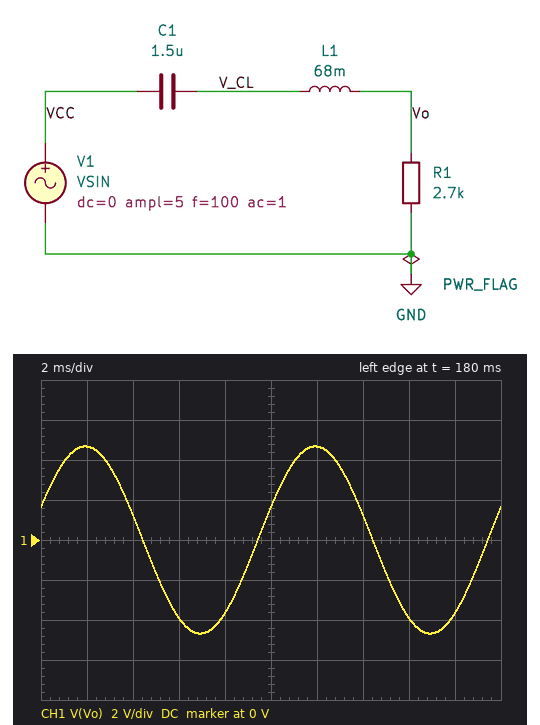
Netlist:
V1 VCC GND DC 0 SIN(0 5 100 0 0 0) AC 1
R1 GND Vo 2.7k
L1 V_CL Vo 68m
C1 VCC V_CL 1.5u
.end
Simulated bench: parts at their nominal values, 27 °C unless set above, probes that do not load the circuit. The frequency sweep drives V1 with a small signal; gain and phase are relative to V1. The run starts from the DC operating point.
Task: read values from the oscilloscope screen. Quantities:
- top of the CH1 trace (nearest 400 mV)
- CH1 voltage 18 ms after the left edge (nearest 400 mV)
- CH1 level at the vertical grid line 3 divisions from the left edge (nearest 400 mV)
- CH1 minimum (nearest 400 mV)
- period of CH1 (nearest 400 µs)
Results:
4.8 V
-3.6 V
-4.0 V
-4.8 V
10.0 ms
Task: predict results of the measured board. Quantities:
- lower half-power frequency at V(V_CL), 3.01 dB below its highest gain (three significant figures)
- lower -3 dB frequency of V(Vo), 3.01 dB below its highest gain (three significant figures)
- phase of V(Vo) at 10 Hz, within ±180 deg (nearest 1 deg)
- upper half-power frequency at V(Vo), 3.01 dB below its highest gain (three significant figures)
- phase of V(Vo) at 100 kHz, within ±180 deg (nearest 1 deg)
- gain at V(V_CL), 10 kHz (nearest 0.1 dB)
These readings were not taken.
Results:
39.5 Hz
39.1 Hz
76 deg
6.36 kHz
-86 deg
0 dB
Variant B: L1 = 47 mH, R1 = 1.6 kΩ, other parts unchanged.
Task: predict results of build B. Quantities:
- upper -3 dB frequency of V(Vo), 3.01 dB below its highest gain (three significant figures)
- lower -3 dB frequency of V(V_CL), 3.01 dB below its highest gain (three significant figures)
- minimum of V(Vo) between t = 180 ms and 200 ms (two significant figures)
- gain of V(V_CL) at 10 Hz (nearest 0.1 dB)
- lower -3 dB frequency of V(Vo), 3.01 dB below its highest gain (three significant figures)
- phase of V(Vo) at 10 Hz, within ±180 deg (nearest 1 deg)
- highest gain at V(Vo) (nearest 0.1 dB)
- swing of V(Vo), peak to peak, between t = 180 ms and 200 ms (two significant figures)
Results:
5.48 kHz
66.9 Hz
-4.2 V
-16.5 dB
65.5 Hz
81 deg
0 dB
8.4 V
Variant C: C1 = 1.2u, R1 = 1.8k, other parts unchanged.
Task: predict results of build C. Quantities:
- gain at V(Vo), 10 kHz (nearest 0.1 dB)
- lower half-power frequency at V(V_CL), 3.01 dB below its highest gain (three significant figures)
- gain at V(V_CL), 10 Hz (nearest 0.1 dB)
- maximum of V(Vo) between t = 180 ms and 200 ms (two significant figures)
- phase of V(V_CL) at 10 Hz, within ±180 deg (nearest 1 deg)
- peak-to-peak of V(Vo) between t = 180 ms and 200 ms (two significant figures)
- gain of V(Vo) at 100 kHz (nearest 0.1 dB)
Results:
-8.2 dB
74.5 Hz
-17.4 dB
4.1 V
82 deg
8.1 V
-27.5 dB
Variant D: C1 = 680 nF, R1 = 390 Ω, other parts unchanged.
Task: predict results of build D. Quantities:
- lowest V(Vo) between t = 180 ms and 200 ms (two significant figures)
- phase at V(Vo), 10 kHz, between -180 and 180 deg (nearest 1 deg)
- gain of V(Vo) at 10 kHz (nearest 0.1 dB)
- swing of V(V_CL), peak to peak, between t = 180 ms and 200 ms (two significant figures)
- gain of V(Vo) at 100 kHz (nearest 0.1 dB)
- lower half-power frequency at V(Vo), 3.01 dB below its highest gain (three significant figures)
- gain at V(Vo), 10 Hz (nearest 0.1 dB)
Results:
-840 mV
-85 deg
-20.8 dB
1.7 V
-40.8 dB
413 Hz
-35.6 dB
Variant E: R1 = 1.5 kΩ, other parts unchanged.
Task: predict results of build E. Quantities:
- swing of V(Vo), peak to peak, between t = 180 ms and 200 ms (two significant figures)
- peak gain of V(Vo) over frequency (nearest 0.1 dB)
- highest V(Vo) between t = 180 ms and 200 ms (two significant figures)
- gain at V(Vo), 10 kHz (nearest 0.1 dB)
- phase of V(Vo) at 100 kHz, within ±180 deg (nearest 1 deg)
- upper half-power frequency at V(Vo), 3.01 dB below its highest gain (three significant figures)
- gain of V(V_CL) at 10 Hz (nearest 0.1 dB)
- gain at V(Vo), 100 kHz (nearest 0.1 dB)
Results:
8.3 V
0 dB
4.1 V
-9.6 dB
-88 deg
3.58 kHz
-17.1 dB
-29.1 dB
